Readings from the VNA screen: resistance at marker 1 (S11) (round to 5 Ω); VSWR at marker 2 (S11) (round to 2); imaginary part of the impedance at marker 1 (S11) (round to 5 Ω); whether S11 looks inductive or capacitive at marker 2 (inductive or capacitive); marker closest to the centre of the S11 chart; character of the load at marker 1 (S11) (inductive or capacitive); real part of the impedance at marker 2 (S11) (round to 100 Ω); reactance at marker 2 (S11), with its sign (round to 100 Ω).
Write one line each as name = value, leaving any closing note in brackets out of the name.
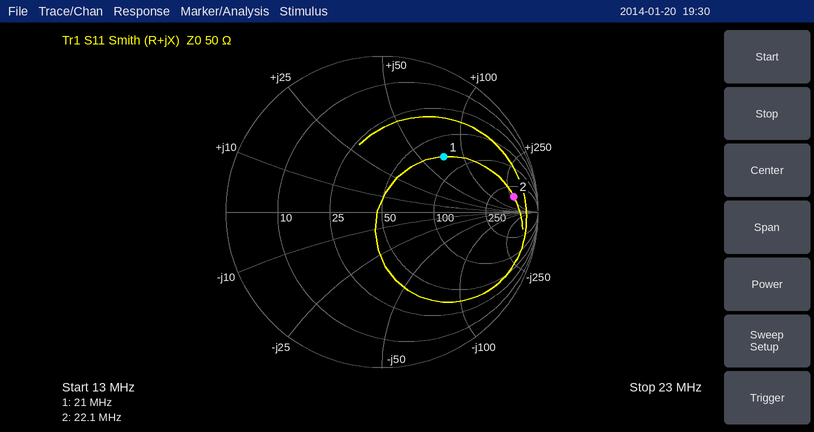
resistance at marker 1 (S11) = 75 Ω
VSWR at marker 2 (S11) = 12
imaginary part of the impedance at marker 1 (S11) = +70 Ω
whether S11 looks inductive or capacitive at marker 2 = inductive
marker closest to the centre of the S11 chart = marker 1
character of the load at marker 1 (S11) = inductive
real part of the impedance at marker 2 (S11) = 400 Ω
reactance at marker 2 (S11), with its sign = +300 Ω
